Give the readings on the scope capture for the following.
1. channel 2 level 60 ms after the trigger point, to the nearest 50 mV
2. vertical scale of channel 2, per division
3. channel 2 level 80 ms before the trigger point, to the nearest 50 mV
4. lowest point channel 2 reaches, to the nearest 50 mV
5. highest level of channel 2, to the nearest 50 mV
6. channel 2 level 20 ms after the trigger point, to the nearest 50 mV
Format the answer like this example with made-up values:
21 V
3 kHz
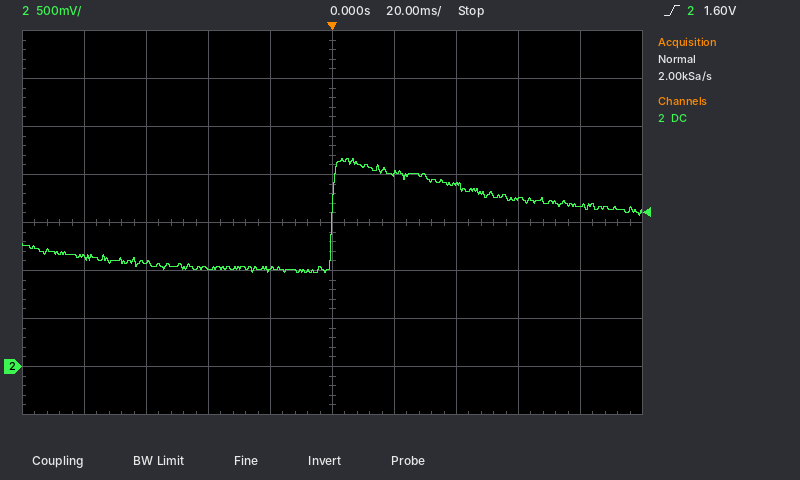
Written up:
1.75 V
500 mV
1.15 V
1.00 V
2.15 V
2.00 V
